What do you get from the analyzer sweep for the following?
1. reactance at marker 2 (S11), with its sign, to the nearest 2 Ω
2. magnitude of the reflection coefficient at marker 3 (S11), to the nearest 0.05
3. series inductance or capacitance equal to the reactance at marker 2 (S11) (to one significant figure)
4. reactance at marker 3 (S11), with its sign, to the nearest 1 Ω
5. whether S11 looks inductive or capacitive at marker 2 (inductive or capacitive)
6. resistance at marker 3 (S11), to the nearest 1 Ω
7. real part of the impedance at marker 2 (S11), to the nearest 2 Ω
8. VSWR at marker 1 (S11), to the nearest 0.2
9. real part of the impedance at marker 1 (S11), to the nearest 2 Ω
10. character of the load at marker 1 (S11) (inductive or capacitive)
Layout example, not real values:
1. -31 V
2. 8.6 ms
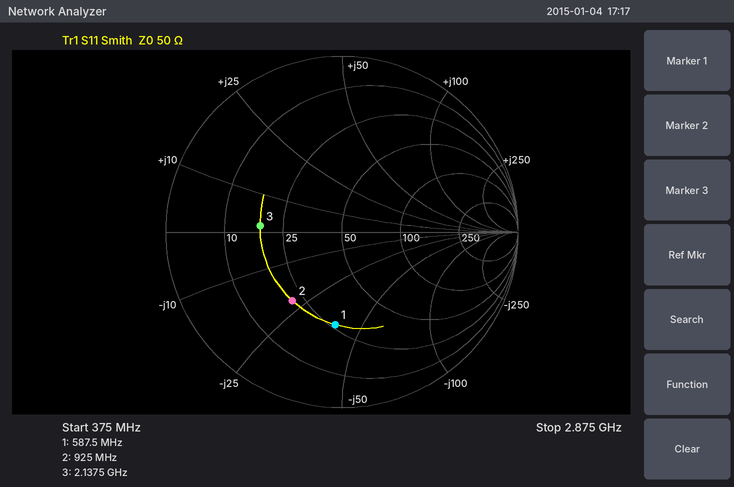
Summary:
1. -22 Ω
2. 0.45
3. 8 pF
4. +2 Ω
5. capacitive
6. 18 Ω
7. 22 Ω
8. 3.2
9. 26 Ω
10. capacitive
